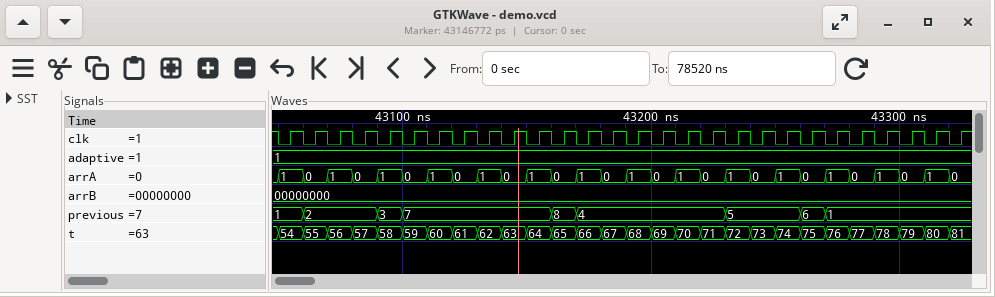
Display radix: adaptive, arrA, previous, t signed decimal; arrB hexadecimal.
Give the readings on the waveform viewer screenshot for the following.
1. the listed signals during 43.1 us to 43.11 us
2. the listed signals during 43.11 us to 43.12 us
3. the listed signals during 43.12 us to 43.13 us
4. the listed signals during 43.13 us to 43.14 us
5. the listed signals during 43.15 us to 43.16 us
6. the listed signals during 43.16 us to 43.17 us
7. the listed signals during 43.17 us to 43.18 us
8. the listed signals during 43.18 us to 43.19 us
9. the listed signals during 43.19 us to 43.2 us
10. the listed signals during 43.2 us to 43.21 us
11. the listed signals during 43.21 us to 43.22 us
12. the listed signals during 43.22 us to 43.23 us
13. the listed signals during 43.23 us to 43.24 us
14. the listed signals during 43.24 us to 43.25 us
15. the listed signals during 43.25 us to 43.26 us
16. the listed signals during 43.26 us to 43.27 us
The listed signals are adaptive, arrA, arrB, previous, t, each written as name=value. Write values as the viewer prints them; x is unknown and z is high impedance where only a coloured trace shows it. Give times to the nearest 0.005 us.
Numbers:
adaptive=1, arrA=0, arrB=00000000, previous=7, t=59
adaptive=1, arrA=1, arrB=00000000, previous=7, t=60
adaptive=1, arrA=0, arrB=00000000, previous=7, t=61
adaptive=1, arrA=1, arrB=00000000, previous=7, t=62
adaptive=1, arrA=1, arrB=00000000, previous=7, t=64
adaptive=1, arrA=0, arrB=00000000, previous=8, t=65
adaptive=1, arrA=1, arrB=00000000, previous=4, t=66
adaptive=1, arrA=0, arrB=00000000, previous=4, t=67
adaptive=1, arrA=1, arrB=00000000, previous=4, t=68
adaptive=1, arrA=0, arrB=00000000, previous=4, t=69
adaptive=1, arrA=1, arrB=00000000, previous=4, t=70
adaptive=1, arrA=0, arrB=00000000, previous=4, t=71
adaptive=1, arrA=1, arrB=00000000, previous=5, t=72
adaptive=1, arrA=0, arrB=00000000, previous=5, t=73
adaptive=1, arrA=1, arrB=00000000, previous=5, t=74
adaptive=1, arrA=0, arrB=00000000, previous=6, t=75
